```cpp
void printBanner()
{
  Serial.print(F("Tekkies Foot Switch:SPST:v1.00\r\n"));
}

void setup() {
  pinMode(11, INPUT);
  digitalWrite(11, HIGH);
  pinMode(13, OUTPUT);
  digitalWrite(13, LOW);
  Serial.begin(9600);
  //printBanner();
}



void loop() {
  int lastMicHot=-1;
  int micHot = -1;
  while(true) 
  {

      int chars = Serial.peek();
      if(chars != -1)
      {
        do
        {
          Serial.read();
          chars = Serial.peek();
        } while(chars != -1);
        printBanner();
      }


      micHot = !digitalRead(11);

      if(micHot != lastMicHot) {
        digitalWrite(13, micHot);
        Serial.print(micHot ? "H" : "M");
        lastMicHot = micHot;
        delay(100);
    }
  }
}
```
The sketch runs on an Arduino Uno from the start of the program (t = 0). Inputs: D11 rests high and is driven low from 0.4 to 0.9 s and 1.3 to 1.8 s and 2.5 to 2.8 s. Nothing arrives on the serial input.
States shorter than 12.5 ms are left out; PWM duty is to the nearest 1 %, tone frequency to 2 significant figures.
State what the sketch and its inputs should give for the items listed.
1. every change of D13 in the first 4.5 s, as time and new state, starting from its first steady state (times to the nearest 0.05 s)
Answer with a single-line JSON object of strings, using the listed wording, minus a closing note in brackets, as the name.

{"every change of D13 in the first 4.5 s, as time and new state, starting from its first steady state": "0 s low; 0.4 s high; 0.9 s low; 1.3 s high; 1.8 s low; 2.5 s high; 2.8 s low"}
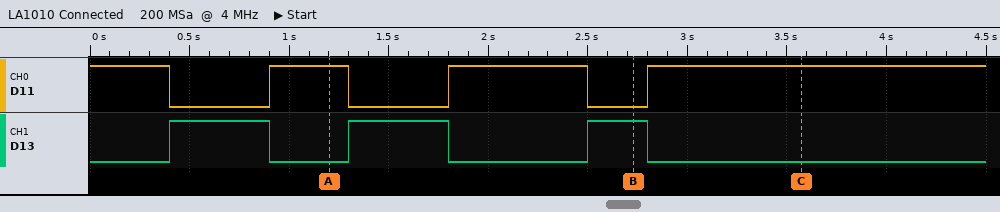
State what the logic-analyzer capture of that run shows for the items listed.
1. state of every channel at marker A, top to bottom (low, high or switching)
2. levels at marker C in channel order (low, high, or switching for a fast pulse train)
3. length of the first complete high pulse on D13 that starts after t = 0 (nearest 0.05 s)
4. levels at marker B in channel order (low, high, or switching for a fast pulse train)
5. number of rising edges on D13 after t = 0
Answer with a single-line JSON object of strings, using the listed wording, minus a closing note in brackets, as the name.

{"state of every channel at marker A, top to bottom": "D11 high, D13 low", "levels at marker C in channel order": "D11 high, D13 low", "length of the first complete high pulse on D13 that starts after t = 0": "0.50 s", "levels at marker B in channel order": "D11 low, D13 high", "number of rising edges on D13 after t = 0": "3"}
